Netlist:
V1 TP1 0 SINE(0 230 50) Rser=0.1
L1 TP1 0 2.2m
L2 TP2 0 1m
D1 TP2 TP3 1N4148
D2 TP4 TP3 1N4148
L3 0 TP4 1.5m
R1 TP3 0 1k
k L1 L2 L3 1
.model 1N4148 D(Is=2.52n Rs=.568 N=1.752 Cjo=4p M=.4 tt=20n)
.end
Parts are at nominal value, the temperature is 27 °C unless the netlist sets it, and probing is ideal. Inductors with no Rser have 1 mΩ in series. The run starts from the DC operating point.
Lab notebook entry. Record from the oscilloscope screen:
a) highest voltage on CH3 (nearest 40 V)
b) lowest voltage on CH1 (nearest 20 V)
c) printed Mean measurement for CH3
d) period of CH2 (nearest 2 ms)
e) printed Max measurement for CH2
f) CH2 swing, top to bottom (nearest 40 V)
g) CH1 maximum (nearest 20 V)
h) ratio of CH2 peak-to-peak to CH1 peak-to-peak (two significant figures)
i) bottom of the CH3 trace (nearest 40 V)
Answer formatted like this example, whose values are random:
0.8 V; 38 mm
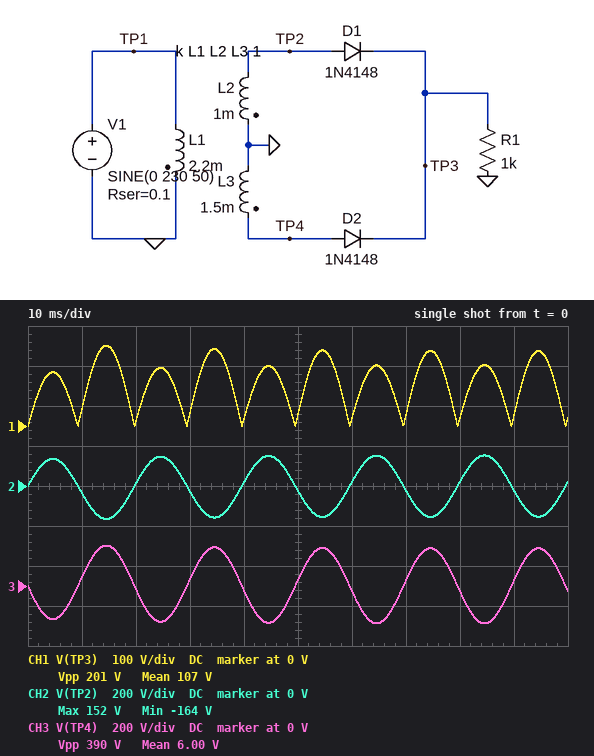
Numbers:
200 V; 0 V; 6.00 V; 20 ms; 152 V; 320 V; 200 V; 1.6; -200 V
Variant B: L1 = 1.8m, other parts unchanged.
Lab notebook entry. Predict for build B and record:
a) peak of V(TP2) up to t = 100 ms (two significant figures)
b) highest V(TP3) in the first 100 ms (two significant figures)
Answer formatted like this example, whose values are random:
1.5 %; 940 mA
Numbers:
170 V; 220 V
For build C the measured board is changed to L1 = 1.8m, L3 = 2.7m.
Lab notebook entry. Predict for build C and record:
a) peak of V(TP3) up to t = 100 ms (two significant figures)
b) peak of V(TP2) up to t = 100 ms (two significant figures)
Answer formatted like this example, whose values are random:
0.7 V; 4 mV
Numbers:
300 V; 170 V
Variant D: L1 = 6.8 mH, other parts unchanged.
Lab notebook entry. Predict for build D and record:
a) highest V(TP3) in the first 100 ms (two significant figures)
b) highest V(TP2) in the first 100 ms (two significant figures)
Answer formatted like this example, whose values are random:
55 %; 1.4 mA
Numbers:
110 V; 87 V
